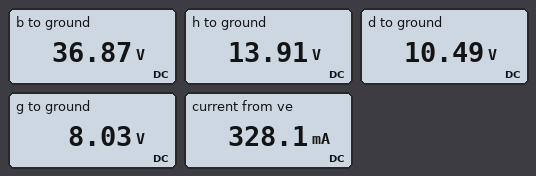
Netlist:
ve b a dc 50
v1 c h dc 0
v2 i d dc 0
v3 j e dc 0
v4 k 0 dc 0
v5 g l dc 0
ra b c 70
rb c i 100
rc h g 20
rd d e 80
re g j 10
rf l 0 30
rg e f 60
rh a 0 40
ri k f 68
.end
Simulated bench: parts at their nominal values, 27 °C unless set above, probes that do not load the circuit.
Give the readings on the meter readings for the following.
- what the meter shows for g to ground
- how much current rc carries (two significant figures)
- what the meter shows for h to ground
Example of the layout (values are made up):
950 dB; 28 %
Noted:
8.03 V; 290 mA; 13.91 V
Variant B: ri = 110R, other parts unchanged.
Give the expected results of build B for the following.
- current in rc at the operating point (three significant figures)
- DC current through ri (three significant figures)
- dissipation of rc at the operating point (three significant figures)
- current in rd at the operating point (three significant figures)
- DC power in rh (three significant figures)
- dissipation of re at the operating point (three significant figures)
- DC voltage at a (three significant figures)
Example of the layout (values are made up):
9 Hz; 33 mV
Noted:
292 mA; 48.1 mA; 1.71 W; 33.3 mA; 4.24 W; 2.19 mW; -13.0 V
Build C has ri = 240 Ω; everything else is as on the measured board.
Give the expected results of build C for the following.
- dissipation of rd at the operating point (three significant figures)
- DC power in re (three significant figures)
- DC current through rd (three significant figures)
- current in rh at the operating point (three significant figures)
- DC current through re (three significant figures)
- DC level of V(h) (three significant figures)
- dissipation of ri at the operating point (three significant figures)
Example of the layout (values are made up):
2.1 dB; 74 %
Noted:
82.3 mW; 73.4 µW; 32.1 mA; 322 mA; 2.71 mA; 14.6 V; 207 mW
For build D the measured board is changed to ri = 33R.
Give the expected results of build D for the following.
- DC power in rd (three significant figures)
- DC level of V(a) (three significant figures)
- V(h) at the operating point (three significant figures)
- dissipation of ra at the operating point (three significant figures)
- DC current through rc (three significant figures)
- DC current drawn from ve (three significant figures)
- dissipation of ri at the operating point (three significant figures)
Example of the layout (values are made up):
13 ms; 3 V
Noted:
99.4 mW; -13.3 V; 13.5 V; 7.69 W; 296 mA; 331 mA; 198 mW
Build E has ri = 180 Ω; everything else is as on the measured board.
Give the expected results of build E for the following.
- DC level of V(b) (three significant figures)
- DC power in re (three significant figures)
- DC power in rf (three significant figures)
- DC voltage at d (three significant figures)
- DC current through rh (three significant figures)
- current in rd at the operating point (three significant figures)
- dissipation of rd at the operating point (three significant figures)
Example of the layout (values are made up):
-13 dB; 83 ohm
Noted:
37.1 V; 109 µW; 2.48 W; 11.2 V; 323 mA; 32.5 mA; 84.5 mW
